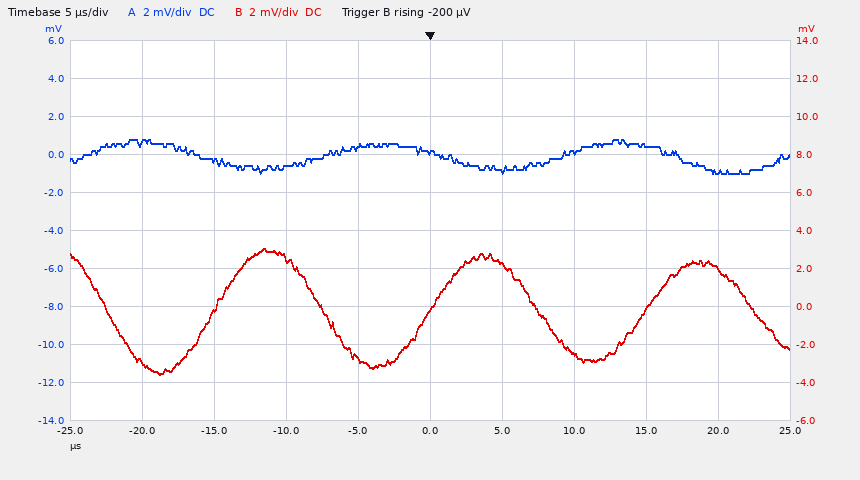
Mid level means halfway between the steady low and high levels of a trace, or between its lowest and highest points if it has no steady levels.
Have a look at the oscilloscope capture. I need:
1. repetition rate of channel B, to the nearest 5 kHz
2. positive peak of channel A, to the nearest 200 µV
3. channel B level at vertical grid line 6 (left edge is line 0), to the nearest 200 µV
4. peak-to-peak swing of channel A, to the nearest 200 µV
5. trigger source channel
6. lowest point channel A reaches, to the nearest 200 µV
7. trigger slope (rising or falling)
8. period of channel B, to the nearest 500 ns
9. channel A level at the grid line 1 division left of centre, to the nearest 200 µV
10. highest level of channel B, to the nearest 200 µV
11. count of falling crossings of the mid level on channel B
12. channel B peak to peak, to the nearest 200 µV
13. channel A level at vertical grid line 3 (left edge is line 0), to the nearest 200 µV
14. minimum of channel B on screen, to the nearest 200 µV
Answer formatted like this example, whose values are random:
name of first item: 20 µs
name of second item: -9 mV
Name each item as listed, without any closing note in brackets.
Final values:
repetition rate of channel B, to the nearest 5 kHz: 65 kHz
positive peak of channel A, to the nearest 200 µV: 800 µV
channel B level at vertical grid line 6 (left edge is line 0), to the nearest 200 µV: 2.2 mV
peak-to-peak swing of channel A, to the nearest 200 µV: 1.8 mV
trigger source channel: channel B
lowest point channel A reaches, to the nearest 200 µV: -1.0 mV
trigger slope: rising
period of channel B, to the nearest 500 ns: 15.0 µs
channel A level at the grid line 1 division left of centre, to the nearest 200 µV: 400 µV
highest level of channel B, to the nearest 200 µV: 3.0 mV
count of falling crossings of the mid level on channel B: 4
channel B peak to peak, to the nearest 200 µV: 6.6 mV
channel A level at vertical grid line 3 (left edge is line 0), to the nearest 200 µV: -600 µV
minimum of channel B on screen, to the nearest 200 µV: -3.6 mV
